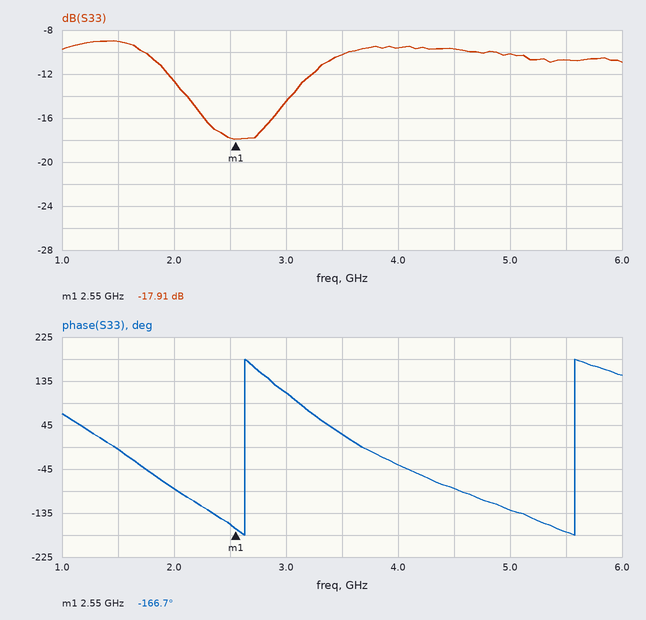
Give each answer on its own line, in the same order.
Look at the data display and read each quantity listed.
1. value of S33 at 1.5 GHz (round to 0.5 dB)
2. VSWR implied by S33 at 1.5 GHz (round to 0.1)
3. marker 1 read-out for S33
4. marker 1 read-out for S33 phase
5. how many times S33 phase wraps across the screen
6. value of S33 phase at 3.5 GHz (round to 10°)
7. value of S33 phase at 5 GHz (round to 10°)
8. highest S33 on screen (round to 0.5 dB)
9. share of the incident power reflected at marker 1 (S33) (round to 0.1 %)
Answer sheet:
-9.0 dB
2.1
-17.91 dB
-166.7°
2
30°
-130°
-9.0 dB
1.6 %
